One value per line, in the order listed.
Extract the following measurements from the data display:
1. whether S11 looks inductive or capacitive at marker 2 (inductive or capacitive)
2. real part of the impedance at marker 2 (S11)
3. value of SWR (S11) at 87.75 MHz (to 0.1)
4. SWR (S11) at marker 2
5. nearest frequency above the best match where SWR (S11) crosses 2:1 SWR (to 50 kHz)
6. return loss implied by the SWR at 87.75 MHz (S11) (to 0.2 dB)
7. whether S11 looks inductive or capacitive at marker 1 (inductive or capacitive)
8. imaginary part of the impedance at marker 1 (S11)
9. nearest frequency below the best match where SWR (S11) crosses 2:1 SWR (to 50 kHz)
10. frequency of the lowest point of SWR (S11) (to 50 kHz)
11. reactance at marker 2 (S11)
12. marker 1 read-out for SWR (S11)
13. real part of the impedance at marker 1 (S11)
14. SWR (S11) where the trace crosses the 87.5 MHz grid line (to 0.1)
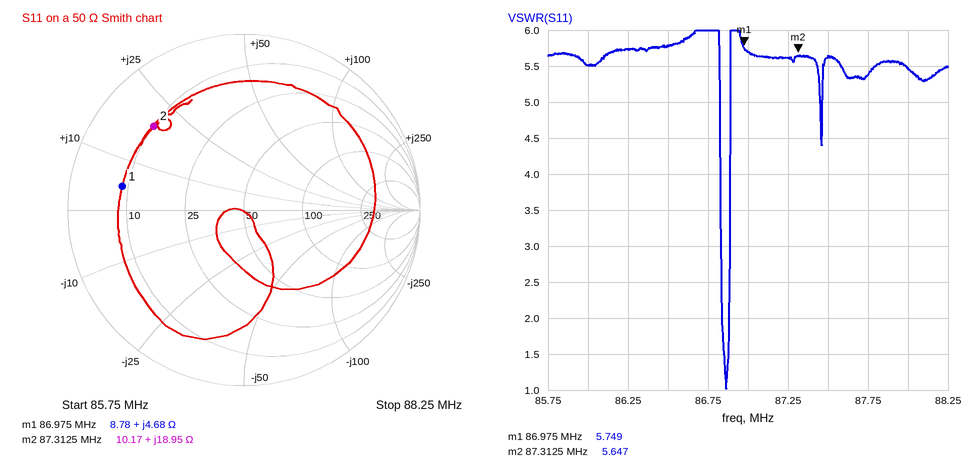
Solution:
inductive
10.17 Ω
5.4
5.647
86.90 MHz
3.2 dB
inductive
+4.68 Ω
86.85 MHz
86.85 MHz
+18.95 Ω
5.749
8.78 Ω
5.6
